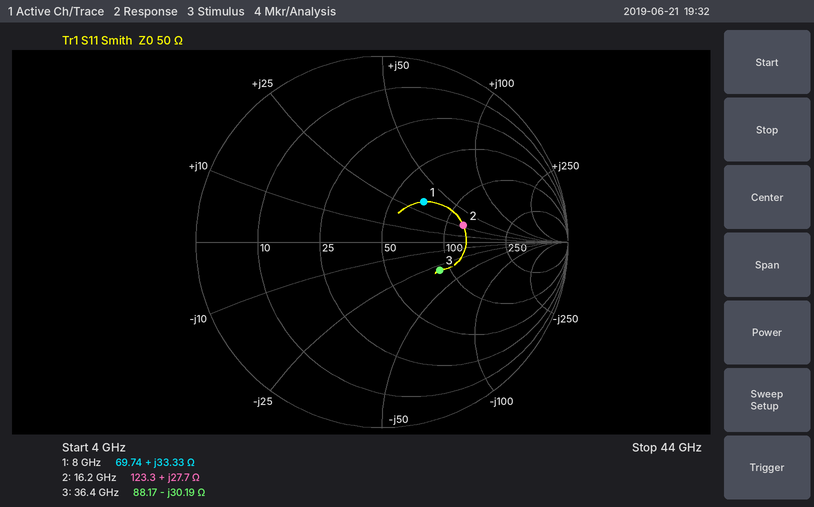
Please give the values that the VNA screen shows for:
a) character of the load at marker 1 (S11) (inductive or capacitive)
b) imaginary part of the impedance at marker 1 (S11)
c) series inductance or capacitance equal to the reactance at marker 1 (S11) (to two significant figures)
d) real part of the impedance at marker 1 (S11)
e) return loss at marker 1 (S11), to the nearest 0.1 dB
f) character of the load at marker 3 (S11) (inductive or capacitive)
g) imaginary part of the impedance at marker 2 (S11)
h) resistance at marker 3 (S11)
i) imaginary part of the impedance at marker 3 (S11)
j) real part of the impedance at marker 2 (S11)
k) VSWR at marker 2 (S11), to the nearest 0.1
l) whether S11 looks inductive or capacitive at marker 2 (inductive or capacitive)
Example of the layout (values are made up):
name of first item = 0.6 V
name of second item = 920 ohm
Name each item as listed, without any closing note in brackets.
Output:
character of the load at marker 1 (S11) = inductive
imaginary part of the impedance at marker 1 = +33.33 Ω
series inductance or capacitance equal to the reactance at marker 1 (S11) = 660 pH
real part of the impedance at marker 1 = 69.74 Ω
return loss at marker 1 (S11), to the nearest 0.1 dB = 10.1 dB
character of the load at marker 3 (S11) = capacitive
imaginary part of the impedance at marker 2 = +27.7 Ω
resistance at marker 3 = 88.17 Ω
imaginary part of the impedance at marker 3 = -30.19 Ω
real part of the impedance at marker 2 = 123.3 Ω
VSWR at marker 2 (S11), to the nearest 0.1 = 2.6
whether S11 looks inductive or capacitive at marker 2 = inductive
